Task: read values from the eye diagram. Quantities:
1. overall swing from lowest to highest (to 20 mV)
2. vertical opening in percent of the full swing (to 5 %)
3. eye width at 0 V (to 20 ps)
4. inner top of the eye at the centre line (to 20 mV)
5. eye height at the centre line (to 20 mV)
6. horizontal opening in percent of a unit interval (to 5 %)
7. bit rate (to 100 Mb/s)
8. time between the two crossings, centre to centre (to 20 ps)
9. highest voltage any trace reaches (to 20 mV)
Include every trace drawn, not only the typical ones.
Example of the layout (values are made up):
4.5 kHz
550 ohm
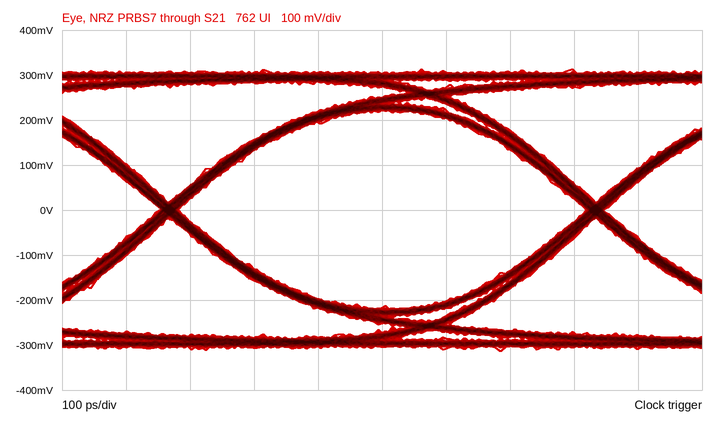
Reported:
620 mV
70 %
640 ps
220 mV
440 mV
95 %
1.5 Gb/s
660 ps
320 mV
